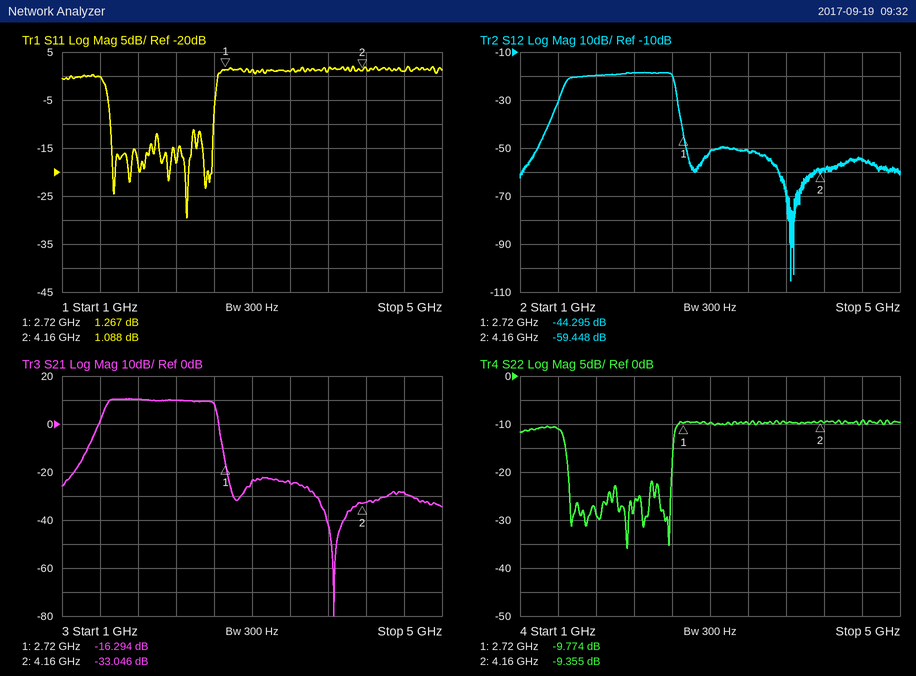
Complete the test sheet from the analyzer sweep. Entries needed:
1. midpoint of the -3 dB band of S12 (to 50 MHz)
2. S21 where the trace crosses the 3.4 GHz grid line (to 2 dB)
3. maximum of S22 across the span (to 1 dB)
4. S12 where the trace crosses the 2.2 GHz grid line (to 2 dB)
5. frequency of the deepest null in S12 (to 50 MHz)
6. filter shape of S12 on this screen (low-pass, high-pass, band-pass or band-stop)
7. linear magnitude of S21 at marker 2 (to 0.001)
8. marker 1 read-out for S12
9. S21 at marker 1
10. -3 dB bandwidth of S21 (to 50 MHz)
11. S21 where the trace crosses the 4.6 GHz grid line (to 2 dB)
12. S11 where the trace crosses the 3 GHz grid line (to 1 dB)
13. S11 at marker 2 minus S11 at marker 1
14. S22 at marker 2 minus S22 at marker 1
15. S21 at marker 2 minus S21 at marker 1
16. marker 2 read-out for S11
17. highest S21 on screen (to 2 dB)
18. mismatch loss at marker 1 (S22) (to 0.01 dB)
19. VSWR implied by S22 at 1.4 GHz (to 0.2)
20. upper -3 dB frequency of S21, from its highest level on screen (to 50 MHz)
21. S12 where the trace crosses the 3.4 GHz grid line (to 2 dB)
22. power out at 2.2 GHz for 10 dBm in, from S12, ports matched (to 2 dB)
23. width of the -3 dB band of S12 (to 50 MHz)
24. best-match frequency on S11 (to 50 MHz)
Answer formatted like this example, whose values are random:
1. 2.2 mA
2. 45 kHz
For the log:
1. 2.05 GHz
2. -24 dB
3. -9 dB
4. -18 dB
5. 3.85 GHz
6. band-pass
7. 0.022
8. -44.295 dB
9. -16.294 dB
10. 1.15 GHz
11. -28 dB
12. 1 dB
13. -0.179 dB
14. 0.419 dB
15. -16.752 dB
16. 1.088 dB
17. 10 dB
18. 0.48 dB
19. 1.8
20. 2.60 GHz
21. -52 dB
22. -8 dBm
23. 1.10 GHz
24. 2.30 GHz
